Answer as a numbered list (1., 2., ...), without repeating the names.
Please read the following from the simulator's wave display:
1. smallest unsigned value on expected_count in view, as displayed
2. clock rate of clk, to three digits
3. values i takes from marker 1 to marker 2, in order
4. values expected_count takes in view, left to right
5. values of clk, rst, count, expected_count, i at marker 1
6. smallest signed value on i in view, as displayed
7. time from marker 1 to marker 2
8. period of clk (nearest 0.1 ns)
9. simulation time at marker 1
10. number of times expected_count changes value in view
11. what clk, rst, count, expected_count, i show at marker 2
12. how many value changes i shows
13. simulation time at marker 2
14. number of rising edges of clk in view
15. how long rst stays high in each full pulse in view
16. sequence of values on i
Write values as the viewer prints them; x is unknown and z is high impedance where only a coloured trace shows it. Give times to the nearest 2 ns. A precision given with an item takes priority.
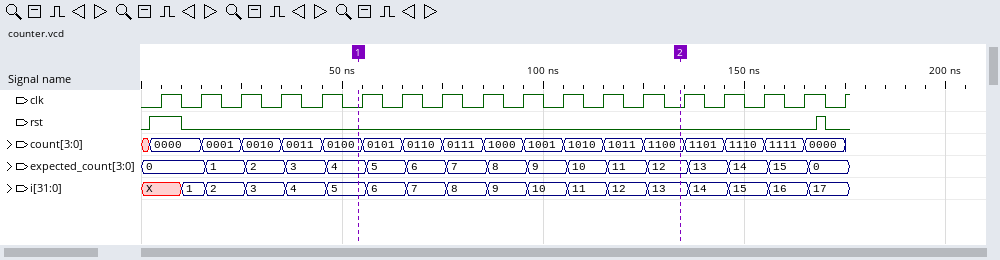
1. 0
2. 100 MHz
3. 5, 6, 7, 8, 9, 10, 11, 12, 13
4. 0, 1, 2, 3, 4, 5, 6, 7, 8, 9, 10, 11, 12, 13, 14, 15, 0
5. clk=0, rst=0, count=0100, expected_count=4, i=5
6. 1
7. 80 ns
8. 10 ns
9. 54 ns
10. 16
11. clk=0, rst=0, count=1100, expected_count=12, i=13
12. 17
13. 134 ns
14. 18
15. 8 ns, 2 ns
16. X, 1, 2, 3, 4, 5, 6, 7, 8, 9, 10, 11, 12, 13, 14, 15, 16, 17
